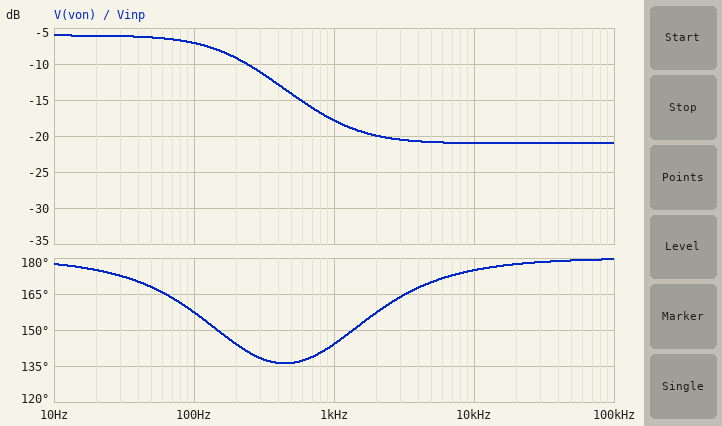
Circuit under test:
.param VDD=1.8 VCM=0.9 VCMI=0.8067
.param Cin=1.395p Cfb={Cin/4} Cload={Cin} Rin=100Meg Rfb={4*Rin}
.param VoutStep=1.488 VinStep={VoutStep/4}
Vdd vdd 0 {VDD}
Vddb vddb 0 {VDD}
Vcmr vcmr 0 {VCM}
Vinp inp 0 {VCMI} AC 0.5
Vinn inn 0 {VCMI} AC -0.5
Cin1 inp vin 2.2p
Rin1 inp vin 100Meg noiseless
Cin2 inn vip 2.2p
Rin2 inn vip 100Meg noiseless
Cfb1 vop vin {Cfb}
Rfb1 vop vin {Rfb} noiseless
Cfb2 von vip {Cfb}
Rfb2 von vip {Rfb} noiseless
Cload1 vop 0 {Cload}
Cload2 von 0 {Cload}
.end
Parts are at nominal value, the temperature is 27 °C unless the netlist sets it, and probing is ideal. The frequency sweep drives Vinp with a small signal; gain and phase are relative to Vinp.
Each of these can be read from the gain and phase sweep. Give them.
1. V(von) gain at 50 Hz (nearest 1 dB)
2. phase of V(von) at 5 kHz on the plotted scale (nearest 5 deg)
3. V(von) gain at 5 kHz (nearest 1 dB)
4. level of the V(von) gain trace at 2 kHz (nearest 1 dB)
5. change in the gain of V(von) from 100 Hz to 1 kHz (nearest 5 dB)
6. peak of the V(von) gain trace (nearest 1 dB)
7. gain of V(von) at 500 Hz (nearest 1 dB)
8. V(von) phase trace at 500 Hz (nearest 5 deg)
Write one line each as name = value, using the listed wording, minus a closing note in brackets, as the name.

V(von) gain at 50 Hz = -6 dB
phase of V(von) at 5 kHz on the plotted scale = 170 deg
V(von) gain at 5 kHz = -21 dB
level of the V(von) gain trace at 2 kHz = -20 dB
change in the gain of V(von) from 100 Hz to 1 kHz = -10 dB
peak of the V(von) gain trace = -6 dB
gain of V(von) at 500 Hz = -14 dB
V(von) phase trace at 500 Hz = 135 deg
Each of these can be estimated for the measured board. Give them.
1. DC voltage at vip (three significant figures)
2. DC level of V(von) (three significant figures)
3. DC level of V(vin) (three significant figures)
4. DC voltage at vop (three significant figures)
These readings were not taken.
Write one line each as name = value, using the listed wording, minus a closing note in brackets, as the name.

DC voltage at vip = 807 mV
DC level of V(von) = 807 mV
DC level of V(vin) = 807 mV
DC voltage at vop = 807 mV
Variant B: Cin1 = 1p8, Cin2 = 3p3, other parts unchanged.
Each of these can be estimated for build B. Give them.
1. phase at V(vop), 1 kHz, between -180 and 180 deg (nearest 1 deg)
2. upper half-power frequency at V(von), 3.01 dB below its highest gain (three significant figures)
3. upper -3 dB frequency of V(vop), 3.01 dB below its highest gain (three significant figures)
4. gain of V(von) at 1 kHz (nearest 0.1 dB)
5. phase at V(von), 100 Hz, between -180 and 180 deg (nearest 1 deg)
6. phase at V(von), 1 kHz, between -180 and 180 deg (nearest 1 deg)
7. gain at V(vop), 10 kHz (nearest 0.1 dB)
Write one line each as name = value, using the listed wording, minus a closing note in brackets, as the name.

phase at V(vop), 1 kHz, between -180 and 180 deg = -37 deg
upper half-power frequency at V(von), 3.01 dB below its highest gain = 192 Hz
upper -3 dB frequency of V(vop), 3.01 dB below its highest gain = 194 Hz
gain of V(von) at 1 kHz = -17.5 dB
phase at V(von), 100 Hz, between -180 and 180 deg = 158 deg
phase at V(von), 1 kHz, between -180 and 180 deg = 145 deg
gain at V(vop), 10 kHz = -15.2 dB
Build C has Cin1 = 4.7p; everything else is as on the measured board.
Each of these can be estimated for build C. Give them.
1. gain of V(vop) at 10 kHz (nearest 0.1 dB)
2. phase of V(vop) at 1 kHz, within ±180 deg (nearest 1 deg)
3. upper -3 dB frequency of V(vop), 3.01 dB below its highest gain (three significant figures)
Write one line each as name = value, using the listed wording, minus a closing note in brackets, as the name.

gain of V(vop) at 10 kHz = -14.4 dB
phase of V(vop) at 1 kHz, within ±180 deg = -35 deg
upper -3 dB frequency of V(vop), 3.01 dB below its highest gain = 191 Hz
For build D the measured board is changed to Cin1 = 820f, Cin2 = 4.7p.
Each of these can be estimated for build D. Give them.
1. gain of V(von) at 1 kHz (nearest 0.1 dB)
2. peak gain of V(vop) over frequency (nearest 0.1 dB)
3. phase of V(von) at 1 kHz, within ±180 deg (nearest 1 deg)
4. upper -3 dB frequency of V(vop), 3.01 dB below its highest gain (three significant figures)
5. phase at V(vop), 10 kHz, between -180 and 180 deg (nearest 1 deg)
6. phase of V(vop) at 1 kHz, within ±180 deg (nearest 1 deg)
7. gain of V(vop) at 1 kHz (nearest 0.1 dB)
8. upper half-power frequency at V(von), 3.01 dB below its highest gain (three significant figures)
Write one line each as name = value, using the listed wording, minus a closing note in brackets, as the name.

gain of V(von) at 1 kHz = -17.3 dB
peak gain of V(vop) over frequency = 0 dB
phase of V(von) at 1 kHz, within ±180 deg = 145 deg
upper -3 dB frequency of V(vop), 3.01 dB below its highest gain = 198 Hz
phase at V(vop), 10 kHz, between -180 and 180 deg = -7 deg
phase of V(vop) at 1 kHz, within ±180 deg = -41 deg
gain of V(vop) at 1 kHz = -12.2 dB
upper half-power frequency at V(von), 3.01 dB below its highest gain = 191 Hz
